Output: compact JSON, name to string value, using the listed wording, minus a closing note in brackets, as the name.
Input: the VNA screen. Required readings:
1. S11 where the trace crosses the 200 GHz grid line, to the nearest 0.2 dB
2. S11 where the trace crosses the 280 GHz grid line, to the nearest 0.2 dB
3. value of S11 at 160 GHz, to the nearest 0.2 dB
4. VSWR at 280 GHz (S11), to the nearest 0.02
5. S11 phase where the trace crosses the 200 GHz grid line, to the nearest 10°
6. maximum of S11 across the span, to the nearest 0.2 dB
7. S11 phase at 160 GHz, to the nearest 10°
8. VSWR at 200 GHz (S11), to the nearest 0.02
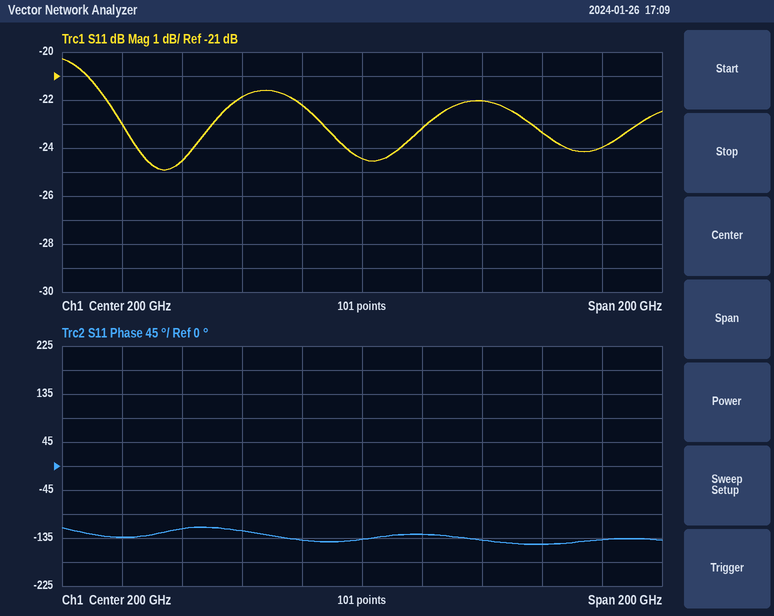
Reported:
{"S11 where the trace crosses the 200 GHz grid line, to the nearest 0.2 dB": "-24.4 dB", "S11 where the trace crosses the 280 GHz grid line, to the nearest 0.2 dB": "-24.0 dB", "value of S11 at 160 GHz, to the nearest 0.2 dB": "-21.8 dB", "VSWR at 280 GHz (S11), to the nearest 0.02": "1.14", "S11 phase where the trace crosses the 200 GHz grid line, to the nearest 10°": "-140°", "maximum of S11 across the span, to the nearest 0.2 dB": "-20.2 dB", "S11 phase at 160 GHz, to the nearest 10°": "-120°", "VSWR at 200 GHz (S11), to the nearest 0.02": "1.12"}
